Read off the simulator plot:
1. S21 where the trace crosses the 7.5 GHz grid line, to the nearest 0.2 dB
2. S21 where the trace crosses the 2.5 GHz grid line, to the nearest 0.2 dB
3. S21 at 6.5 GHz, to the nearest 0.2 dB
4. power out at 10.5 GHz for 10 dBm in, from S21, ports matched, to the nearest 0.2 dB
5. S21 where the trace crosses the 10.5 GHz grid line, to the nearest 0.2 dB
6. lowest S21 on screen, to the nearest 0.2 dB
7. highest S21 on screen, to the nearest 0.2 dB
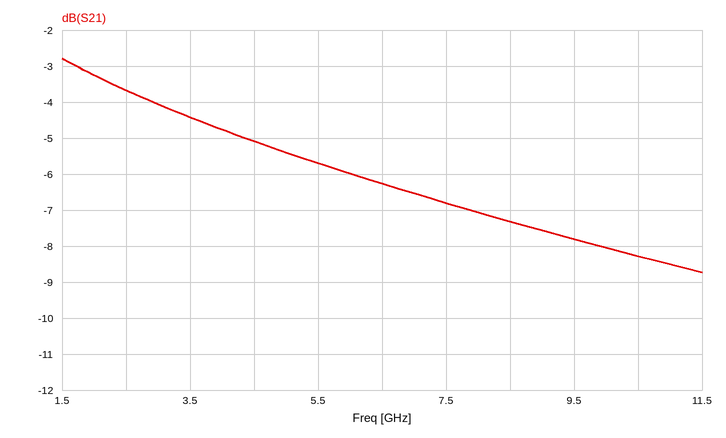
-6.8 dB
-3.6 dB
-6.2 dB
1.8 dBm
-8.2 dB
-8.8 dB
-2.8 dB
